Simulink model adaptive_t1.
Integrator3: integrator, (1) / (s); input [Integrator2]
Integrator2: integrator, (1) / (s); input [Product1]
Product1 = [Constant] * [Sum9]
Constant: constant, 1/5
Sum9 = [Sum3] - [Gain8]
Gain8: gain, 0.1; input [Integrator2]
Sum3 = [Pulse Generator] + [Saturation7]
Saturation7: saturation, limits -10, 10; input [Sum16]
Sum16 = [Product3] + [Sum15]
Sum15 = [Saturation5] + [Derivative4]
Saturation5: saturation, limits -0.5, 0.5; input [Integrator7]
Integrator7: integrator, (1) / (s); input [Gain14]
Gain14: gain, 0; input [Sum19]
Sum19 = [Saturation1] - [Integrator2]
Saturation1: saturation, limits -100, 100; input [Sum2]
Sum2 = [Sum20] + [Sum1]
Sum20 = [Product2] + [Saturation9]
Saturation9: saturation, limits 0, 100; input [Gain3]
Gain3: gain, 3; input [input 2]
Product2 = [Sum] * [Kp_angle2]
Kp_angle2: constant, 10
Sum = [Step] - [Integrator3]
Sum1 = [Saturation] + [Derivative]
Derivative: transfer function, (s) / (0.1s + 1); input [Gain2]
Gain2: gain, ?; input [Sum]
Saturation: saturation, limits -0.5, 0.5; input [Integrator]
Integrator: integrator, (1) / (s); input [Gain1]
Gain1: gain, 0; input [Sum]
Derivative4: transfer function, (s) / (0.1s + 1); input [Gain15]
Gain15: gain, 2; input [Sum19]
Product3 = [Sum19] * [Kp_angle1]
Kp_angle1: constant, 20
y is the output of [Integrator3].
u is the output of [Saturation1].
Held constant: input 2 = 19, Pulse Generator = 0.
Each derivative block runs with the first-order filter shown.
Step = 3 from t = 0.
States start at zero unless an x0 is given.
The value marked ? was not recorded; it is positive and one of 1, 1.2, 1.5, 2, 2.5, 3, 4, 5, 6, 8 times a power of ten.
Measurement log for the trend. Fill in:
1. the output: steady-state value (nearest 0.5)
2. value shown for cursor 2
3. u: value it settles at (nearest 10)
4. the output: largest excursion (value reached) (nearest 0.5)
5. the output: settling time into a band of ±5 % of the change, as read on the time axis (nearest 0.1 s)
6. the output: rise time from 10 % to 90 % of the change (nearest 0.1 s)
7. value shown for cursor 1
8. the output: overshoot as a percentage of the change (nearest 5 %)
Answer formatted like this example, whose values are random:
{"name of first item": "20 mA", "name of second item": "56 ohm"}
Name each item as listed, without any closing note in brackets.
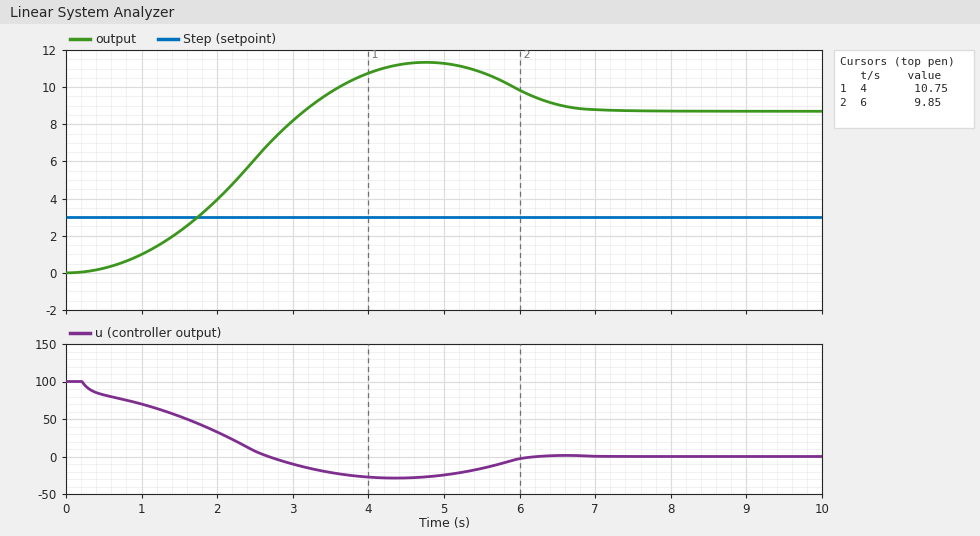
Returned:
{"the output: steady-state value": "8.5", "value shown for cursor 2": "9.85", "u: value it settles at": "0", "the output: largest excursion (value reached)": "11.5", "the output: settling time into a band of ±5 % of the change, as read on the time axis": "6.4 s", "the output: rise time from 10 % to 90 % of the change": "2.0 s", "value shown for cursor 1": "10.75", "the output: overshoot as a percentage of the change": "30 %"}
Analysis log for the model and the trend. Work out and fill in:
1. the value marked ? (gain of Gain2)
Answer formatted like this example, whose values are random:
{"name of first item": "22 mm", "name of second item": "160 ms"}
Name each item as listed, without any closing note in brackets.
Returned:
{"the value marked ?": "4"}
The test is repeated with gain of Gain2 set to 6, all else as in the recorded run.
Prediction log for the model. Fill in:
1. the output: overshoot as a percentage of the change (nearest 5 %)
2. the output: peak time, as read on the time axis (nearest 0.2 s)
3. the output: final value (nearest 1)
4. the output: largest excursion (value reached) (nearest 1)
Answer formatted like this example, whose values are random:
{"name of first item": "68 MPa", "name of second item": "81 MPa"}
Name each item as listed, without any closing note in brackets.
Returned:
{"the output: overshoot as a percentage of the change": "15 %", "the output: peak time, as read on the time axis": "4.4 s", "the output: final value": "9", "the output: largest excursion (value reached)": "10"}
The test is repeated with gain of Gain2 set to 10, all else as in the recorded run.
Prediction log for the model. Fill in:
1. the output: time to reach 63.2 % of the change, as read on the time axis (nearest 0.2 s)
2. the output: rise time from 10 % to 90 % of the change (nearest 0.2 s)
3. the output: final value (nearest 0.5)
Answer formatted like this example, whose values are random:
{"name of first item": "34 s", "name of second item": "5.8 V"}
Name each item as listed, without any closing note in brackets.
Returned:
{"the output: time to reach 63.2 % of the change, as read on the time axis": "2.4 s", "the output: rise time from 10 % to 90 % of the change": "2.8 s", "the output: final value": "8.5"}
